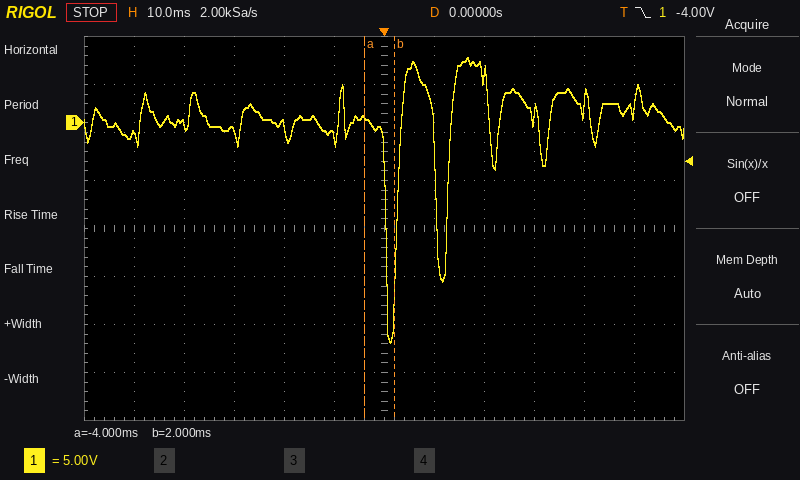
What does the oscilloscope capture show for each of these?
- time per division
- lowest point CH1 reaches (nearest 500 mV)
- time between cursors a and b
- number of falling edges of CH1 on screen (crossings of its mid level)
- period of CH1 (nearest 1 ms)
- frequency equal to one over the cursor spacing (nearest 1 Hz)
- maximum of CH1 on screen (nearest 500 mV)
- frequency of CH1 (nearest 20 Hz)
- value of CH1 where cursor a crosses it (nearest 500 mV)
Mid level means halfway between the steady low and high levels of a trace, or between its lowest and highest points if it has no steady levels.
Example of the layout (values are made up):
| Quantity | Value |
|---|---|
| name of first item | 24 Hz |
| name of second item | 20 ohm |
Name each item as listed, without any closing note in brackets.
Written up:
| Quantity | Value |
|---|---|
| time per division | 10 ms |
| lowest point CH1 reaches | -23.0 V |
| time between cursors a and b | 6 ms |
| number of falling edges of CH1 on screen | 2 |
| period of CH1 | 10 ms |
| frequency equal to one over the cursor spacing | 167 Hz |
| maximum of CH1 on screen | 7.0 V |
| frequency of CH1 | 100 Hz |
| value of CH1 where cursor a crosses it | 500 mV |
